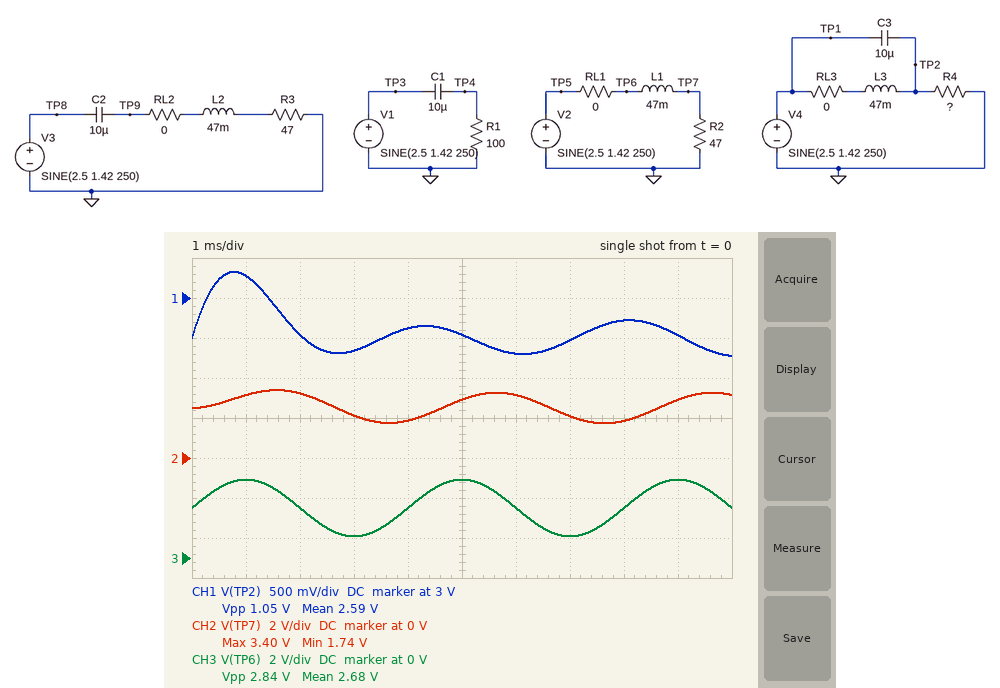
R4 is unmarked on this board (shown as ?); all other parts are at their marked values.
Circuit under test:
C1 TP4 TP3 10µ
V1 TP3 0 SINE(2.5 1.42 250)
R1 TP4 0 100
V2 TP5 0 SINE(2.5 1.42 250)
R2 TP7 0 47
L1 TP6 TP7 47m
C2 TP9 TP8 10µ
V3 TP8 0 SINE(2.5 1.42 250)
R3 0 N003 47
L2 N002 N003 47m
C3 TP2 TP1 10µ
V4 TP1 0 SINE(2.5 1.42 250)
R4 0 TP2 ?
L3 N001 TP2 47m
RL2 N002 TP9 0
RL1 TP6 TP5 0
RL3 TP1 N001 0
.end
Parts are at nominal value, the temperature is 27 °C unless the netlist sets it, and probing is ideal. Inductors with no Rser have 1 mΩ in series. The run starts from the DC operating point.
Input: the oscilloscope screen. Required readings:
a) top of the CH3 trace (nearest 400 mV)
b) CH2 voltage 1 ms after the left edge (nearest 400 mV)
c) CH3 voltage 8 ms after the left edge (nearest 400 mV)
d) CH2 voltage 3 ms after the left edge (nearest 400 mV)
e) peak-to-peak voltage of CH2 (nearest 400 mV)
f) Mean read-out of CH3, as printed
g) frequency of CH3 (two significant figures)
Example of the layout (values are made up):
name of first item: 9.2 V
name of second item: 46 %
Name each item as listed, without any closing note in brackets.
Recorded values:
top of the CH3 trace: 4.0 V
CH2 voltage 1 ms after the left edge: 3.2 V
CH3 voltage 8 ms after the left edge: 2.4 V
CH2 voltage 3 ms after the left edge: 2.0 V
peak-to-peak voltage of CH2: 1.6 V
Mean read-out of CH3, as printed: 2.68 V
frequency of CH3: 250 Hz
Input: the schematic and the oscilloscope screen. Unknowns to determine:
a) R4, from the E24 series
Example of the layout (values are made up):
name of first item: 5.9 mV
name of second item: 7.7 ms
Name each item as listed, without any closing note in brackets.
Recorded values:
R4, from the E24 series: 75 Ω
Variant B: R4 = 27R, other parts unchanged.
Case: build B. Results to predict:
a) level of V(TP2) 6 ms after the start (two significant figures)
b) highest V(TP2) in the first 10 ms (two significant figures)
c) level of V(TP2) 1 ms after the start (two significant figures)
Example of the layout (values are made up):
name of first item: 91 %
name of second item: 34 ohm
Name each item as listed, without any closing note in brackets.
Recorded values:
level of V(TP2) 6 ms after the start: 2.4 V
highest V(TP2) in the first 10 ms: 3.0 V
level of V(TP2) 1 ms after the start: 2.9 V
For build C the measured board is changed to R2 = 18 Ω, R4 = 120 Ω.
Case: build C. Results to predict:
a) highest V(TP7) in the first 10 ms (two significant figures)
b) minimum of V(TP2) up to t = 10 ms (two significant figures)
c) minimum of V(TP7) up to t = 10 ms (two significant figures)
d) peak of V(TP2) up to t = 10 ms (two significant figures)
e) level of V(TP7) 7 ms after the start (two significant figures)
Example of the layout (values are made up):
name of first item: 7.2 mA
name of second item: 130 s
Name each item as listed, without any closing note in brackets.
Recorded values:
highest V(TP7) in the first 10 ms: 3.0 V
minimum of V(TP2) up to t = 10 ms: 2.1 V
minimum of V(TP7) up to t = 10 ms: 2.2 V
peak of V(TP2) up to t = 10 ms: 3.5 V
level of V(TP7) 7 ms after the start: 2.4 V
